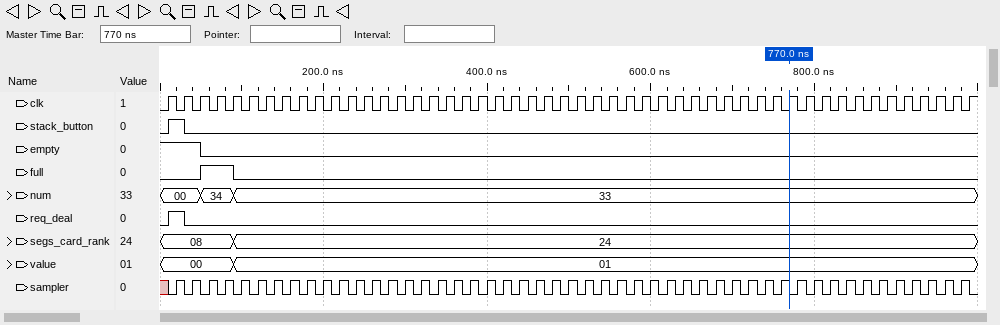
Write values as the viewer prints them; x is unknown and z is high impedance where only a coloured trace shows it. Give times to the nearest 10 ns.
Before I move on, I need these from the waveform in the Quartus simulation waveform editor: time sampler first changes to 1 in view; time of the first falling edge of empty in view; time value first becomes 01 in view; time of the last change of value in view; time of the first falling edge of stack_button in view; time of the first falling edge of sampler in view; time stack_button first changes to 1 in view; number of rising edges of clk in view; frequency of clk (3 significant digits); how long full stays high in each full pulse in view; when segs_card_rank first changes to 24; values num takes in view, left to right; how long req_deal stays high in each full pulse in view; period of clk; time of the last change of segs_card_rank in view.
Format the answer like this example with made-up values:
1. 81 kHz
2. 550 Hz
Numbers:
1. 20 ns
2. 50 ns
3. 90 ns
4. 90 ns
5. 30 ns
6. 30 ns
7. 10 ns
8. 50
9. 50.0 MHz
10. 40 ns
11. 90 ns
12. 00, 34, 33
13. 20 ns
14. 20 ns
15. 90 ns
